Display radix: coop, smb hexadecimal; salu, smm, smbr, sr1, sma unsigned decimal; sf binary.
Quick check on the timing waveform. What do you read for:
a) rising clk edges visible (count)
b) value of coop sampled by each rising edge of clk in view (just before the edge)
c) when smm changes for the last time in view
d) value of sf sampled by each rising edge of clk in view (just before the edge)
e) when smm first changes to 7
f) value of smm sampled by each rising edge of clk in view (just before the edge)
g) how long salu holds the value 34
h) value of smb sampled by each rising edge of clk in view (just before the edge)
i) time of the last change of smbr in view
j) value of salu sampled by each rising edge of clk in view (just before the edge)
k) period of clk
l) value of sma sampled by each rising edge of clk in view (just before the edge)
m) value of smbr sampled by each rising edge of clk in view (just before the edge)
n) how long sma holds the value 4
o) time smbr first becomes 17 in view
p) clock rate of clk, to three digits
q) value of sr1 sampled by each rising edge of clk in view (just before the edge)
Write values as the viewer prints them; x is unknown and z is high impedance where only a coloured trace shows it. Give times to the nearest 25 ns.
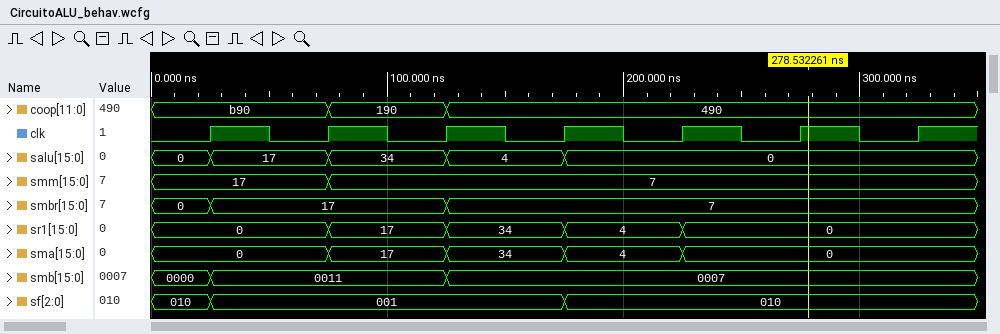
7
b90, b90, 190, 490, 490, 490, 490
75 ns
010, 001, 001, 001, 010, 010, 010
75 ns
17, 17, 7, 7, 7, 7, 7
50 ns
0000, 0011, 0011, 0007, 0007, 0007, 0007
125 ns
0, 17, 34, 4, 0, 0, 0
50 ns
0, 0, 17, 34, 4, 0, 0
0, 17, 17, 7, 7, 7, 7
50 ns
25 ns
20.0 MHz
0, 0, 17, 34, 4, 0, 0
